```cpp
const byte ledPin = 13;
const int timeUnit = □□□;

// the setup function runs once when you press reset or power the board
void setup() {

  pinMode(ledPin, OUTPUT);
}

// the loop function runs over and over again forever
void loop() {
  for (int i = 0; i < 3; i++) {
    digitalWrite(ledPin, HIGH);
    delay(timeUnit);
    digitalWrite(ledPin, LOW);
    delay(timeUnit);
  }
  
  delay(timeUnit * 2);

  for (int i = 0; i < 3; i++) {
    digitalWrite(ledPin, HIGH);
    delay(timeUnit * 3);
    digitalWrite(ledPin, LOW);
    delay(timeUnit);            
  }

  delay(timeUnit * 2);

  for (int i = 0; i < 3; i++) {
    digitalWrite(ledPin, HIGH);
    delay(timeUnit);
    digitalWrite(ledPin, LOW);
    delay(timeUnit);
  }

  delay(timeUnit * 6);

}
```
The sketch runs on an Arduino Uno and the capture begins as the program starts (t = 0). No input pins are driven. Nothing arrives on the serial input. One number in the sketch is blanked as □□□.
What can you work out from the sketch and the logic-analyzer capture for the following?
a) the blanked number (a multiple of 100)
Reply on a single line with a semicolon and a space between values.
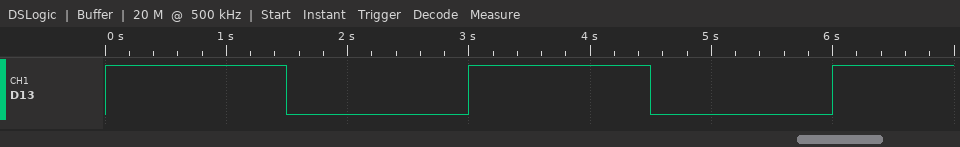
1500
